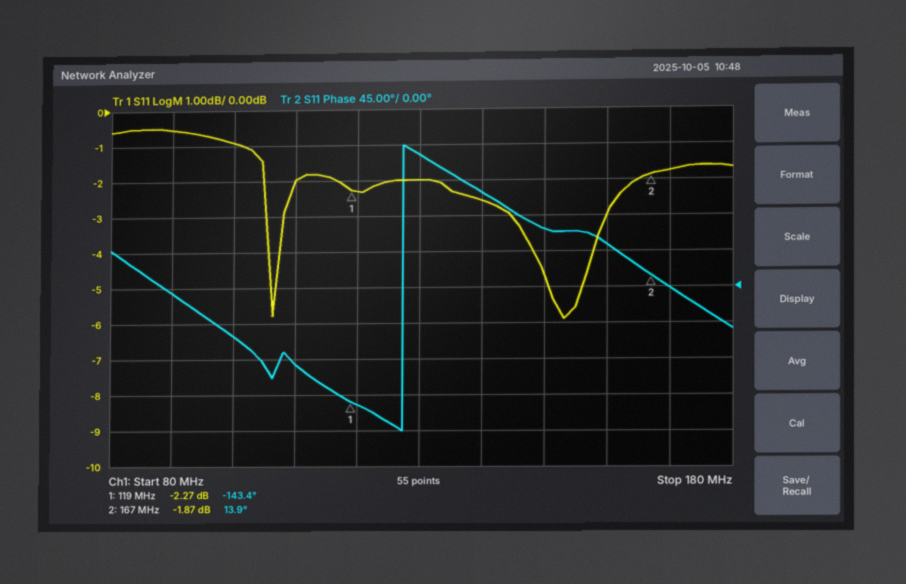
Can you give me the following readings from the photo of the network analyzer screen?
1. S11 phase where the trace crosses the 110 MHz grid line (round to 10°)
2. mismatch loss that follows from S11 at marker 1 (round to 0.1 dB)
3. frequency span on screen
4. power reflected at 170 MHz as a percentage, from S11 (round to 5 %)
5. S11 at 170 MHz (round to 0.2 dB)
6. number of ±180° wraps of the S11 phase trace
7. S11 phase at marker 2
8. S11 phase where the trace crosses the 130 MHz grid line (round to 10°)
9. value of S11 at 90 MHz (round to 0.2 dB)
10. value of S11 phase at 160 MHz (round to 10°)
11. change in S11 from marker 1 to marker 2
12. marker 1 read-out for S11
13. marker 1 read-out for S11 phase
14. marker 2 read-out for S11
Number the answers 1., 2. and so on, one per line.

1. -100°
2. 3.9 dB
3. 100 MHz
4. 65 %
5. -1.8 dB
6. 1
7. 13.9°
8. 170°
9. -0.6 dB
10. 50°
11. 0.40 dB
12. -2.27 dB
13. -143.4°
14. -1.87 dB
